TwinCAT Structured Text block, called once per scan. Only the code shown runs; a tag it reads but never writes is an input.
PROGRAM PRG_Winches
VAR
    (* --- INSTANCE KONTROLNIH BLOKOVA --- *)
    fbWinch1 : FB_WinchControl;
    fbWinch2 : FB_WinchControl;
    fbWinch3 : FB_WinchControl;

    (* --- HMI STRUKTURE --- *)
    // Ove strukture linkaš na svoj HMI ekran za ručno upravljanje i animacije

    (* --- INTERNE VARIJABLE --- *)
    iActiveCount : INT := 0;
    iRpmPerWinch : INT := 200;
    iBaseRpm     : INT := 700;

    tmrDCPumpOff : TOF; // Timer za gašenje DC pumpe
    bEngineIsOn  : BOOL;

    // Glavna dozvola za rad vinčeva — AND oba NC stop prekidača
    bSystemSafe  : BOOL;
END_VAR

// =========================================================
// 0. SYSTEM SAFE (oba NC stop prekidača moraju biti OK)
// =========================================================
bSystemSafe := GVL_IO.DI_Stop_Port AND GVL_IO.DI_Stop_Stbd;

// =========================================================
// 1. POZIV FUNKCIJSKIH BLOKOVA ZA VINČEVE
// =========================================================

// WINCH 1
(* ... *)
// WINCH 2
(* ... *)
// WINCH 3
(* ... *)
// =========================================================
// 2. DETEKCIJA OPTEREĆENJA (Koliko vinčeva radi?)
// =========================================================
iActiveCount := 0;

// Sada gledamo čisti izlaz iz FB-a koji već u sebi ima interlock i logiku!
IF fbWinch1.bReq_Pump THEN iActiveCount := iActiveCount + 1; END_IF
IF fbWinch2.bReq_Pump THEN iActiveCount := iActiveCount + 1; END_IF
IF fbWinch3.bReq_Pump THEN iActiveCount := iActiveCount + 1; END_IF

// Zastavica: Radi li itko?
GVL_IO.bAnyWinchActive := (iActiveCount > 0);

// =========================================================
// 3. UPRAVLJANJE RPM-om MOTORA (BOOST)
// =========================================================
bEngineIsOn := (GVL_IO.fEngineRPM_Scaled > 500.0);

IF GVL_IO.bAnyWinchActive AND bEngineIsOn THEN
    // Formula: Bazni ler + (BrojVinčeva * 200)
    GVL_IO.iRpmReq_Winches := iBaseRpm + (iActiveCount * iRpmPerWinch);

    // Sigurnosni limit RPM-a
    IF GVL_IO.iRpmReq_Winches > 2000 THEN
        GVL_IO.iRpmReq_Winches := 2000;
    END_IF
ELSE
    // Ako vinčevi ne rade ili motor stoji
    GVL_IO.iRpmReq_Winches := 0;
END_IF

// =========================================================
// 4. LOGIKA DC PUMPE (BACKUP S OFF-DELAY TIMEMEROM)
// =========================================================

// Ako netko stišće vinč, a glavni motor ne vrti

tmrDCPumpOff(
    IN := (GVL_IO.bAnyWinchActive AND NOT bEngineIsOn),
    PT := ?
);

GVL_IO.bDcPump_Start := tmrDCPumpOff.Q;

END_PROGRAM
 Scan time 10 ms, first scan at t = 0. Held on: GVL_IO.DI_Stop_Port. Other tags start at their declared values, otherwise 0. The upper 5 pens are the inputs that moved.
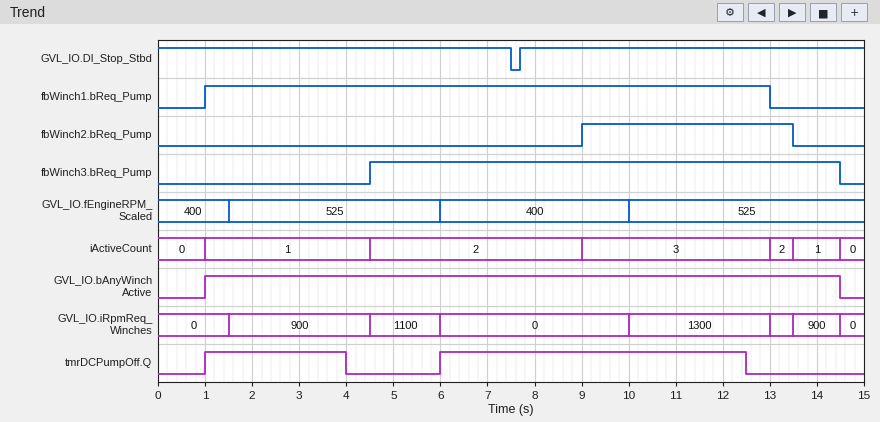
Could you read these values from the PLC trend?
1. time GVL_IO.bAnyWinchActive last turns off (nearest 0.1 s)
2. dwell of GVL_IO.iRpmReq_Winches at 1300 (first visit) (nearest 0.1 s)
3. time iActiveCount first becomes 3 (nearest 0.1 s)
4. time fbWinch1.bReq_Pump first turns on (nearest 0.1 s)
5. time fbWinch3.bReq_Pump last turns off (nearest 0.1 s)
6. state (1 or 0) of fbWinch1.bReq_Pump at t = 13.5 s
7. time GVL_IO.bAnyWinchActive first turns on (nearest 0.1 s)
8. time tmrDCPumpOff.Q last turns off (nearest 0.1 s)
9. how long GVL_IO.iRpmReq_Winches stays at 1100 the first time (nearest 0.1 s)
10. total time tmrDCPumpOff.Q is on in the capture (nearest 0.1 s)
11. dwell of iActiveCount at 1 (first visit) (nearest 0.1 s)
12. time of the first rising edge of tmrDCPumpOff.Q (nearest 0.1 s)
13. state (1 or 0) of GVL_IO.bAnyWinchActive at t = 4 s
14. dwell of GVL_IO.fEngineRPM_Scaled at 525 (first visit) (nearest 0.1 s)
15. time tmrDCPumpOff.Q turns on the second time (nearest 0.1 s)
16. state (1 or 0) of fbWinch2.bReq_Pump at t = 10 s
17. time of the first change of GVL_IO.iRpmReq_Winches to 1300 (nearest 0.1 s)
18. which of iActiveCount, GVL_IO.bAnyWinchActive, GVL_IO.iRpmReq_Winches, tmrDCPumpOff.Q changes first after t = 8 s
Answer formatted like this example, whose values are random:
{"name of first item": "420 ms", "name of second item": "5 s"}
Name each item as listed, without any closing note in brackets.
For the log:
{"time GVL_IO.bAnyWinchActive last turns off": "14.5 s", "dwell of GVL_IO.iRpmReq_Winches at 1300 (first visit)": "3.0 s", "time iActiveCount first becomes 3": "9.0 s", "time fbWinch1.bReq_Pump first turns on": "1.0 s", "time fbWinch3.bReq_Pump last turns off": "14.5 s", "state (1 or 0) of fbWinch1.bReq_Pump at t = 13.5 s": "0", "time GVL_IO.bAnyWinchActive first turns on": "1.0 s", "time tmrDCPumpOff.Q last turns off": "12.5 s", "how long GVL_IO.iRpmReq_Winches stays at 1100 the first time": "1.5 s", "total time tmrDCPumpOff.Q is on in the capture": "9.5 s", "dwell of iActiveCount at 1 (first visit)": "3.5 s", "time of the first rising edge of tmrDCPumpOff.Q": "1.0 s", "state (1 or 0) of GVL_IO.bAnyWinchActive at t = 4 s": "1", "dwell of GVL_IO.fEngineRPM_Scaled at 525 (first visit)": "4.5 s", "time tmrDCPumpOff.Q turns on the second time": "6.0 s", "state (1 or 0) of fbWinch2.bReq_Pump at t = 10 s": "1", "time of the first change of GVL_IO.iRpmReq_Winches to 1300": "10.0 s", "which of iActiveCount, GVL_IO.bAnyWinchActive, GVL_IO.iRpmReq_Winches, tmrDCPumpOff.Q changes first after t = 8 s": "iActiveCount"}
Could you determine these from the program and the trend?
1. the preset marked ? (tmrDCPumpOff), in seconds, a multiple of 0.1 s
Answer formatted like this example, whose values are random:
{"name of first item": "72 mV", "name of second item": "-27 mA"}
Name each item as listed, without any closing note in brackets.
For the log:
{"the preset marked ? (tmrDCPumpOff), in seconds, a multiple of 0.1 s": "2.5 s"}
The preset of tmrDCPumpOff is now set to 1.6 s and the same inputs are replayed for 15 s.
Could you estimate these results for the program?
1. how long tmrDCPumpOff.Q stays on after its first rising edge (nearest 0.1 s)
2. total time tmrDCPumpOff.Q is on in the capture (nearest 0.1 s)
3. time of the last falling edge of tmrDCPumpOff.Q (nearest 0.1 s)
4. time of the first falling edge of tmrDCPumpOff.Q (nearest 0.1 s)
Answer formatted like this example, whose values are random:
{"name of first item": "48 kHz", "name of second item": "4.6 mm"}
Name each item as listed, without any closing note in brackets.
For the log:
{"how long tmrDCPumpOff.Q stays on after its first rising edge": "2.1 s", "total time tmrDCPumpOff.Q is on in the capture": "7.7 s", "time of the last falling edge of tmrDCPumpOff.Q": "11.6 s", "time of the first falling edge of tmrDCPumpOff.Q": "3.1 s"}
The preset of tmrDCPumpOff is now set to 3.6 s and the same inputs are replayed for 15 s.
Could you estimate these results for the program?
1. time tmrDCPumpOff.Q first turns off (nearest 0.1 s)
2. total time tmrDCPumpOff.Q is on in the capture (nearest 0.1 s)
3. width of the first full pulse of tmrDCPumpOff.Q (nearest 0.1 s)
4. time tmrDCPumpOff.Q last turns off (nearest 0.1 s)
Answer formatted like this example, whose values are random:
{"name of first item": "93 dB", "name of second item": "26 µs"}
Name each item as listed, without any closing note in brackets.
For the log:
{"time tmrDCPumpOff.Q first turns off": "5.1 s", "total time tmrDCPumpOff.Q is on in the capture": "11.7 s", "width of the first full pulse of tmrDCPumpOff.Q": "4.1 s", "time tmrDCPumpOff.Q last turns off": "13.6 s"}
